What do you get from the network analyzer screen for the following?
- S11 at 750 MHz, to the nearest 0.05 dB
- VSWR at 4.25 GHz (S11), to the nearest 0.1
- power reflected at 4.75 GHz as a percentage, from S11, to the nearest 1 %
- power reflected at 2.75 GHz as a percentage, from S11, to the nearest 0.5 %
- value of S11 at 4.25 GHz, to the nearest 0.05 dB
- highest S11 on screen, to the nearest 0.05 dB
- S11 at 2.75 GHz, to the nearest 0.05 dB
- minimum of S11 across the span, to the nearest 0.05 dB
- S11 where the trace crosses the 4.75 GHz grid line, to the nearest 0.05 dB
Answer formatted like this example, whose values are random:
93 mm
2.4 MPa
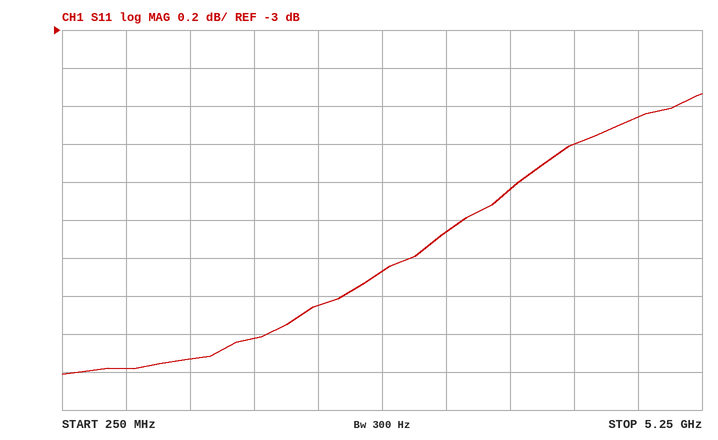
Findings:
-4.80 dB
4.9
45 %
37.5 %
-3.60 dB
-3.35 dB
-4.25 dB
-4.80 dB
-3.45 dB
